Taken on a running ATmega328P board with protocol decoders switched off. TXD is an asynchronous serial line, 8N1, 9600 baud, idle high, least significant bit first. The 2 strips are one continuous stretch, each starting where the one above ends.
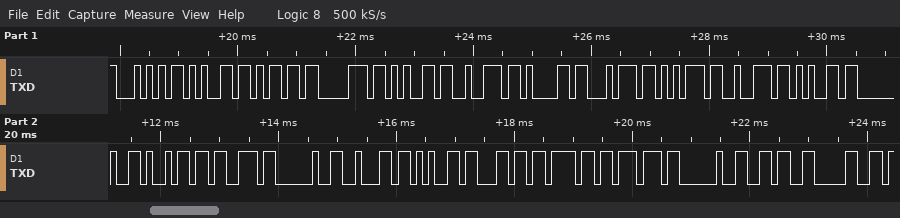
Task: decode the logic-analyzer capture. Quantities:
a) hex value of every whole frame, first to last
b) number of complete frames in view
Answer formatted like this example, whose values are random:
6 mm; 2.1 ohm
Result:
0x54 0x65 0x6D 0x70 0x65 0x72 0x61 0x74 0x75 0x72 0x65 0x20 0x69 0x73 0x20 0x62 0x65 0x6C 0x6F 0x77 0x20 0x36 0x30; 23
